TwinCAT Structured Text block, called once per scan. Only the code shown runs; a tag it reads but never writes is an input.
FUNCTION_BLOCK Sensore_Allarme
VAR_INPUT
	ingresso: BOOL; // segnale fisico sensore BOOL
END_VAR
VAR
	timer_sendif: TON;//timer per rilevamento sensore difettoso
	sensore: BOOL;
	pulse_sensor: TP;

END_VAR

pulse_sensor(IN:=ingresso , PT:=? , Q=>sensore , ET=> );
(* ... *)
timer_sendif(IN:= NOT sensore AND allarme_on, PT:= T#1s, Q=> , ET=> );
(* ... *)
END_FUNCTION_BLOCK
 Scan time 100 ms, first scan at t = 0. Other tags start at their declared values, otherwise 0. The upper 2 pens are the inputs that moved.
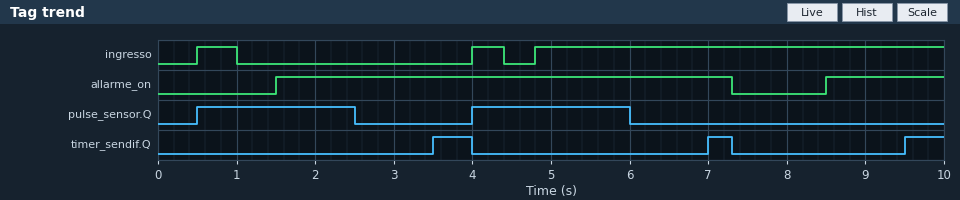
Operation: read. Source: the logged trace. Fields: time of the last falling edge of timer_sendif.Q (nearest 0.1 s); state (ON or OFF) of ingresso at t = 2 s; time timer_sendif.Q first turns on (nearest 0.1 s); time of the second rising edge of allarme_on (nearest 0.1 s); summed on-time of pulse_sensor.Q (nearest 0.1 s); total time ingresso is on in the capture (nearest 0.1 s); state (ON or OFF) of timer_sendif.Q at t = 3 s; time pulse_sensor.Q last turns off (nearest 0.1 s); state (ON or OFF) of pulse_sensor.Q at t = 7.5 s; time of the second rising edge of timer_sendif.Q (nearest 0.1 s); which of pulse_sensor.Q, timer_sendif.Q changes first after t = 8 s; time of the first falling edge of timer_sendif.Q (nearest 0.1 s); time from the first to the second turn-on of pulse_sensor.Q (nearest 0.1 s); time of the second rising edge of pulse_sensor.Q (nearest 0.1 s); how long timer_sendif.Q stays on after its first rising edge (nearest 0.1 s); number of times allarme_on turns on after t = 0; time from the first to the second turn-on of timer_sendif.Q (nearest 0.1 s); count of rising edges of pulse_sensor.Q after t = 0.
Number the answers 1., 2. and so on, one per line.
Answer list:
1. 7.3 s
2. OFF
3. 3.5 s
4. 8.5 s
5. 4.0 s
6. 6.1 s
7. OFF
8. 6.0 s
9. OFF
10. 7.0 s
11. timer_sendif.Q
12. 4.0 s
13. 3.5 s
14. 4.0 s
15. 0.5 s
16. 2
17. 3.5 s
18. 2
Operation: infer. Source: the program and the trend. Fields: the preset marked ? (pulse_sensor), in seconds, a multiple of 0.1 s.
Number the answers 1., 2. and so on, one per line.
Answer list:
1. 2.0 s
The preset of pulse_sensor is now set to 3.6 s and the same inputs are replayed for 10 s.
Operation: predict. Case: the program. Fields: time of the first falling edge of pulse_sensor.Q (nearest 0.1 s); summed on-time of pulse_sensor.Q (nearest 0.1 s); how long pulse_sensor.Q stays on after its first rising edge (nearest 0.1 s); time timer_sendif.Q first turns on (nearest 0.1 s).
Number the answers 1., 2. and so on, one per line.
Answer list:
1. 4.1 s
2. 7.2 s
3. 3.6 s
4. 9.5 s
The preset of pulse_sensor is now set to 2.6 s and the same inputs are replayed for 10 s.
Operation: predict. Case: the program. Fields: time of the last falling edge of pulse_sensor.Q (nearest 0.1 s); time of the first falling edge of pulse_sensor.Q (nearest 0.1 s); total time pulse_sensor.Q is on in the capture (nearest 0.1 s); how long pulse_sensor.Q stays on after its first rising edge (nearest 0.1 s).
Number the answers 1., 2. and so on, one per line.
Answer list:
1. 6.6 s
2. 3.1 s
3. 5.2 s
4. 2.6 s
